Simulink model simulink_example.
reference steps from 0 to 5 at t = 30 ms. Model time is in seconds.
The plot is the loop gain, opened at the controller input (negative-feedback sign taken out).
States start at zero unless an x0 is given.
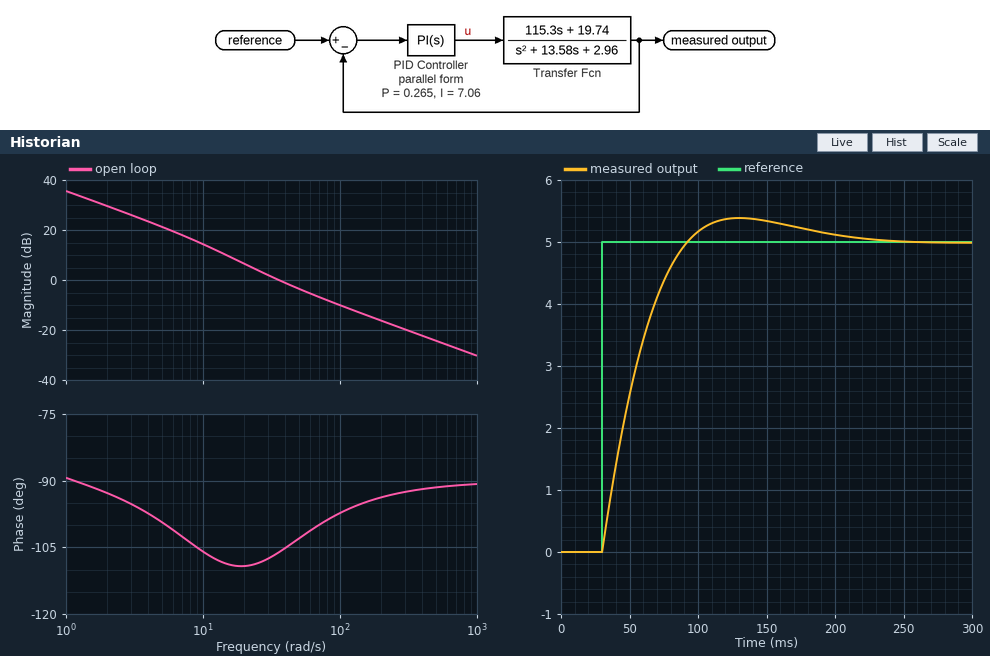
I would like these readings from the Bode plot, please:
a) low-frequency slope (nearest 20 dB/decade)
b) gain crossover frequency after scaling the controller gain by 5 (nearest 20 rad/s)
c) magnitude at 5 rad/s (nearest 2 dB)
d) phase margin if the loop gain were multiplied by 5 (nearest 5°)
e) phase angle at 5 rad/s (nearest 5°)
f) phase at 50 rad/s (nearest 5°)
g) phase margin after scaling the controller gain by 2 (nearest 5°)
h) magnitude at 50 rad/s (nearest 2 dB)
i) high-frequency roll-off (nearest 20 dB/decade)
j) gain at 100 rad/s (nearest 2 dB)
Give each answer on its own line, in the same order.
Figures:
-20 dB/decade
160 rad/s
22 dB
85°
-100°
-105°
80°
-4 dB
-20 dB/decade
-10 dB
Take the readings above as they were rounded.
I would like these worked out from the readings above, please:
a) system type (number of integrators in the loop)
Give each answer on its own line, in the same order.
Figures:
1
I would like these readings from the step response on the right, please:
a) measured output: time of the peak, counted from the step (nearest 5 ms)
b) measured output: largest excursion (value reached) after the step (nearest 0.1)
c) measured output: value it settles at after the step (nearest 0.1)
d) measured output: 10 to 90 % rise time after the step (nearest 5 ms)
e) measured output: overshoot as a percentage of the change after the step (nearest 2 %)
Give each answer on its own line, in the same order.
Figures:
100 ms
5.4
5.0
45 ms
8 %
